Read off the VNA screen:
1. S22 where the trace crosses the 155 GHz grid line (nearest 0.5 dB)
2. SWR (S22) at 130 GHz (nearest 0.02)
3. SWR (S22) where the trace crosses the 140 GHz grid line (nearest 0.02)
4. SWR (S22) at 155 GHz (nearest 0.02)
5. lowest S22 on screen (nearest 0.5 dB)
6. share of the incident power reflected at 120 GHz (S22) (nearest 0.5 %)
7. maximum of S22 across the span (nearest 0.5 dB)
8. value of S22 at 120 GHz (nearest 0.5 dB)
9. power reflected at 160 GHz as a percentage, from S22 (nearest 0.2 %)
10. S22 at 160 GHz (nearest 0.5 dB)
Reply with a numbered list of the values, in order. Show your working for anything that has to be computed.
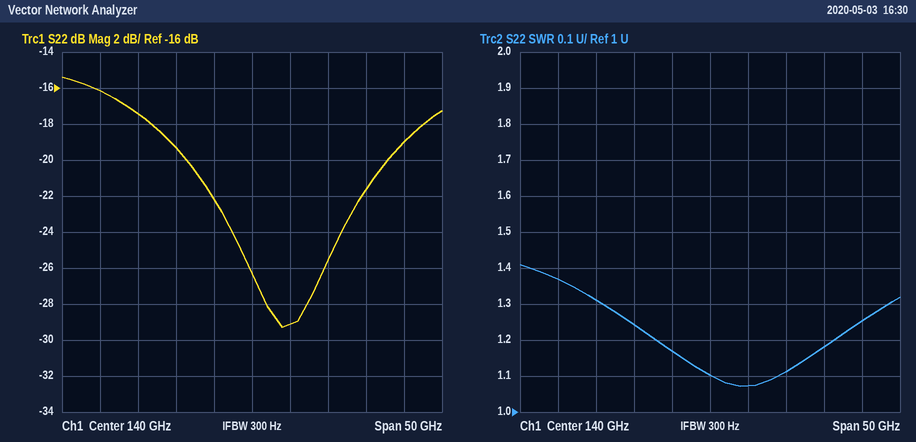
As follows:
1. -21.5 dB
2. 1.24
3. 1.10
4. 1.18
5. -29.5 dB
6. 10^(-16/10) ≈ 2.5 %
7. -15.5 dB
8. -16.0 dB
9. 10^(-19/10) ≈ 1.26 %, so 1.2 % to the nearest 0.2 %
10. -19.0 dB
